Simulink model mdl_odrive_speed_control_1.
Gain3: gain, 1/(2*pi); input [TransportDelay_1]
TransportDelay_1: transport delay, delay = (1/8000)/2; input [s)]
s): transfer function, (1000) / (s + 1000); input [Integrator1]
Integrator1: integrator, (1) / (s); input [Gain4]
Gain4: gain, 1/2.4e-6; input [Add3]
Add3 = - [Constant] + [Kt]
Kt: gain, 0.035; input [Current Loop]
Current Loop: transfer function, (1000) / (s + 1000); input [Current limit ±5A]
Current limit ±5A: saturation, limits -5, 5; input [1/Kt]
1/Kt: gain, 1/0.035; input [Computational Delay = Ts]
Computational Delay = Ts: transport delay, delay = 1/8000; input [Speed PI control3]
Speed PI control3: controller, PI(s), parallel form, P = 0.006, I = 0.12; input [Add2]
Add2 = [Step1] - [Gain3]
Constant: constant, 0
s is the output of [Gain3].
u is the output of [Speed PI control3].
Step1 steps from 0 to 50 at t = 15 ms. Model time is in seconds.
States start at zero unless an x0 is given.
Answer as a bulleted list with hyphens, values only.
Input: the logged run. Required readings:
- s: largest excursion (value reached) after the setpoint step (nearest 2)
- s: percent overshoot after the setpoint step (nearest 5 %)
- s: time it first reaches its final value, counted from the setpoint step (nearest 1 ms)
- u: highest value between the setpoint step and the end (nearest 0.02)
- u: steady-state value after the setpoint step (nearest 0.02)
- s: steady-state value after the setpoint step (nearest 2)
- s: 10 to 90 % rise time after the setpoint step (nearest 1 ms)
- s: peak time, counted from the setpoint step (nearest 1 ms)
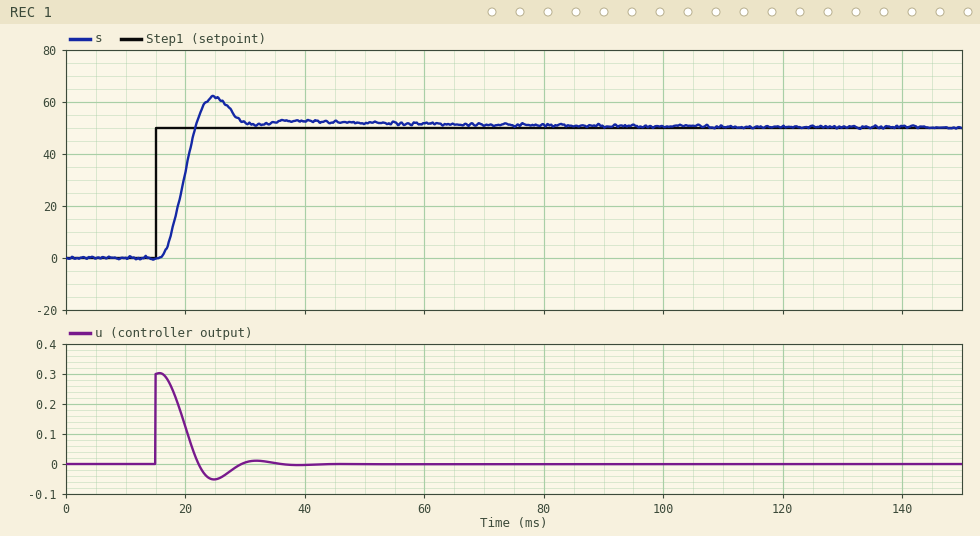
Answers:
- 62
- 25 %
- 7 ms
- 0.30
- 0.00
- 50
- 4 ms
- 10 ms
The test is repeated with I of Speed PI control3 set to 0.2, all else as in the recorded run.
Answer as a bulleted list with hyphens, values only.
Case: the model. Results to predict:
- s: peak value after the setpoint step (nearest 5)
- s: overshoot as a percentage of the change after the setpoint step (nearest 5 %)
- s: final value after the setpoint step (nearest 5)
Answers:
- 65
- 30 %
- 50
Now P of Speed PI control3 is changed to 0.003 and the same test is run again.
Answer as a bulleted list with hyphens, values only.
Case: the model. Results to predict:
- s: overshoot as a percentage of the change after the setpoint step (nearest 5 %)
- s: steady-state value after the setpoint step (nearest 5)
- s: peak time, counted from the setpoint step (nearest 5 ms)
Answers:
- 20 %
- 50
- 15 ms
